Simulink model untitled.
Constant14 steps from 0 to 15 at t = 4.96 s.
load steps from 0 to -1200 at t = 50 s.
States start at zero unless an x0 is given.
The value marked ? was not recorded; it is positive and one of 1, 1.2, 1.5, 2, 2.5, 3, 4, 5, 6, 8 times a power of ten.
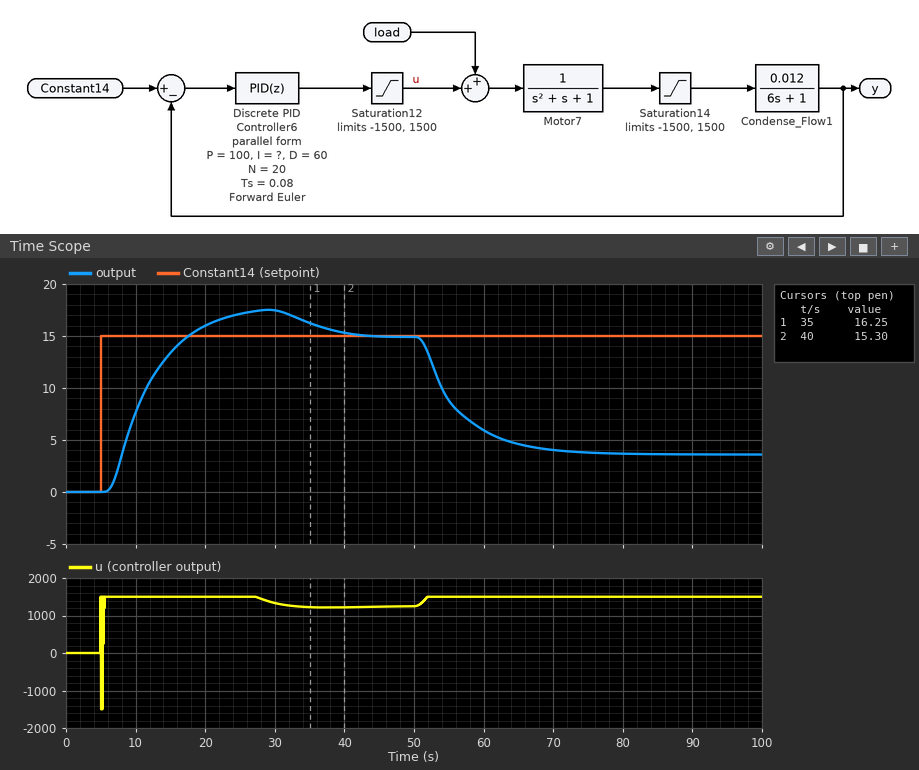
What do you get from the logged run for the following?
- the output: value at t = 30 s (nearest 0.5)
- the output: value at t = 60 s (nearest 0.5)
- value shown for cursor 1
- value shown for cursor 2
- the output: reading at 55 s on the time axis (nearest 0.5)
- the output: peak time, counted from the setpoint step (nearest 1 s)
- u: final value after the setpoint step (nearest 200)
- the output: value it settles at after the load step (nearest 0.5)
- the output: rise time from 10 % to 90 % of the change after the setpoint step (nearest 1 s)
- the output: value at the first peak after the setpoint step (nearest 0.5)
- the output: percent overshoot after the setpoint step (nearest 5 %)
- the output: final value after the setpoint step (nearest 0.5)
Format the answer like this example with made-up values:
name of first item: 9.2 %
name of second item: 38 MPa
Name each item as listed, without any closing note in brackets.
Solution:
the output: value at t = 30 s: 17.5
the output: value at t = 60 s: 6.0
value shown for cursor 1: 16.25
value shown for cursor 2: 15.30
the output: reading at 55 s on the time axis: 9.0
the output: peak time, counted from the setpoint step: 24 s
u: final value after the setpoint step: 1200
the output: value it settles at after the load step: 3.5
the output: rise time from 10 % to 90 % of the change after the setpoint step: 8 s
the output: value at the first peak after the setpoint step: 17.5
the output: percent overshoot after the setpoint step: 15 %
the output: final value after the setpoint step: 15.0
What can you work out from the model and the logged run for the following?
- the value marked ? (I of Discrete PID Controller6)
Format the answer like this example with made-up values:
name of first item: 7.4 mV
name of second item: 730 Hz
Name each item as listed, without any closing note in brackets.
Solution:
the value marked ?: 25
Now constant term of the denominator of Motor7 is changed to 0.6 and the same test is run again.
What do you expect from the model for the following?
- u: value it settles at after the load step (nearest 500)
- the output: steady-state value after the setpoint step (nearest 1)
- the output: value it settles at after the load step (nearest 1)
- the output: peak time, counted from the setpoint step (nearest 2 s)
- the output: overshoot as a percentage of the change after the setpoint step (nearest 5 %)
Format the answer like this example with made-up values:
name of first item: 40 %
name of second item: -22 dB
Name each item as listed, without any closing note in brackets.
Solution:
u: value it settles at after the load step: 1500
the output: steady-state value after the setpoint step: 15
the output: value it settles at after the load step: 6
the output: peak time, counted from the setpoint step: 32 s
the output: overshoot as a percentage of the change after the setpoint step: 20 %
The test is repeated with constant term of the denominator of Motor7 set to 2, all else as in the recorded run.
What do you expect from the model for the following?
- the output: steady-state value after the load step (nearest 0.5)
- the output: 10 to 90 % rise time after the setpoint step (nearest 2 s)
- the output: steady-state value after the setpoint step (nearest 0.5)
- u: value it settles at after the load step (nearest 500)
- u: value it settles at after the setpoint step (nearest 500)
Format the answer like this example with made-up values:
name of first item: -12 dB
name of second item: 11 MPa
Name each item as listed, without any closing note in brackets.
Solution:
the output: steady-state value after the load step: 2.0
the output: 10 to 90 % rise time after the setpoint step: 12 s
the output: steady-state value after the setpoint step: 9.0
u: value it settles at after the load step: 1500
u: value it settles at after the setpoint step: 1500
